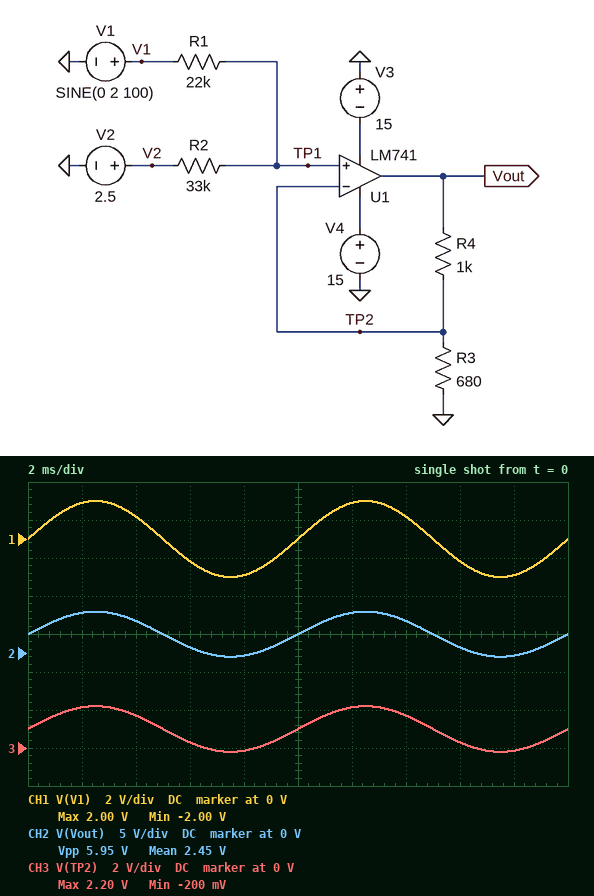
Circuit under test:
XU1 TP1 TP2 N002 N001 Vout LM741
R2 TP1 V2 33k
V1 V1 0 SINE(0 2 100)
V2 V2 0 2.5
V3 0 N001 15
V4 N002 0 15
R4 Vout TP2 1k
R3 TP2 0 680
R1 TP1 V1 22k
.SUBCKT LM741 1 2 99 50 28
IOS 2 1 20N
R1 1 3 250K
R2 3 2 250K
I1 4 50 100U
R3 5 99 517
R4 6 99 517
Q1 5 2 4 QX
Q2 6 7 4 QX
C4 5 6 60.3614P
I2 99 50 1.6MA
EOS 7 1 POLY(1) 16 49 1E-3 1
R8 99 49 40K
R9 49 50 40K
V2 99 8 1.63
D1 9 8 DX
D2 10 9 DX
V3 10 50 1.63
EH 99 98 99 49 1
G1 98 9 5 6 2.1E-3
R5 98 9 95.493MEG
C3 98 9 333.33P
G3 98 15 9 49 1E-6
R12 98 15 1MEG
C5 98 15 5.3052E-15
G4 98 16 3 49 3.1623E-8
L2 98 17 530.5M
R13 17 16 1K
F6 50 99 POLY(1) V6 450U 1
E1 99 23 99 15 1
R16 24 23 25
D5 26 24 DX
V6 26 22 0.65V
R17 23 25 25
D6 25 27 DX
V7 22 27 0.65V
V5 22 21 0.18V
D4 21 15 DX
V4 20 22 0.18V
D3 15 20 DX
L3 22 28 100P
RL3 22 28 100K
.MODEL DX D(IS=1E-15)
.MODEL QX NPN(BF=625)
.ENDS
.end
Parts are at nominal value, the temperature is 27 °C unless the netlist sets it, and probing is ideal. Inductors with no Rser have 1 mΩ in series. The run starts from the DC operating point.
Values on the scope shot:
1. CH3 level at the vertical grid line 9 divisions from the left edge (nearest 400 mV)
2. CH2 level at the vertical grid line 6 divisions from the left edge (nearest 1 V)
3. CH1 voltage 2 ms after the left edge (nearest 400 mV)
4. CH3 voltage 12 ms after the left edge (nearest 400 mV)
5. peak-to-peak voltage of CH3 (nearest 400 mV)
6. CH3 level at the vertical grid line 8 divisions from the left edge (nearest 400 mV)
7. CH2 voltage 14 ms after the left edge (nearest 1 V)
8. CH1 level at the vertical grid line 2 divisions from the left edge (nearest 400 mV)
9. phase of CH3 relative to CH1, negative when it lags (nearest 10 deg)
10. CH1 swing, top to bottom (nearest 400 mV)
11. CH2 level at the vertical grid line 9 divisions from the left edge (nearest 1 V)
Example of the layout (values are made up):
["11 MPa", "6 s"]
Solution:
["0 V", "5 V", "2.0 V", "2.0 V", "2.4 V", "400 mV", "4 V", "1.2 V", "0 deg", "4.0 V", "0 V"]
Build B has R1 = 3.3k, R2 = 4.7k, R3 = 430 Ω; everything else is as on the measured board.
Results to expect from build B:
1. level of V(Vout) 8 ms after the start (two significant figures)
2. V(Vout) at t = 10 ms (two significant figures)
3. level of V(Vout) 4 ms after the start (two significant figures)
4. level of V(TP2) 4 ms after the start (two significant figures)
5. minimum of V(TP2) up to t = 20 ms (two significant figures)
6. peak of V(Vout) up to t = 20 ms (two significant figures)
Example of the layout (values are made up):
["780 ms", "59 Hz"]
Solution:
["-280 mV", "3.4 V", "5.7 V", "1.7 V", "-140 mV", "7.3 V"]
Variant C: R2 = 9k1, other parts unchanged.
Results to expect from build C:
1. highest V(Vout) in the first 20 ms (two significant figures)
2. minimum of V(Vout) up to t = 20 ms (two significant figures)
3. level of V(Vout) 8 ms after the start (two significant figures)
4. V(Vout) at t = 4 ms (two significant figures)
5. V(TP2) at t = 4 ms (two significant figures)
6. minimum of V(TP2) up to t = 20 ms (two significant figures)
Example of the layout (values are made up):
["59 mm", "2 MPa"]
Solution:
["5.8 V", "2.9 V", "3.0 V", "5.2 V", "2.1 V", "1.2 V"]
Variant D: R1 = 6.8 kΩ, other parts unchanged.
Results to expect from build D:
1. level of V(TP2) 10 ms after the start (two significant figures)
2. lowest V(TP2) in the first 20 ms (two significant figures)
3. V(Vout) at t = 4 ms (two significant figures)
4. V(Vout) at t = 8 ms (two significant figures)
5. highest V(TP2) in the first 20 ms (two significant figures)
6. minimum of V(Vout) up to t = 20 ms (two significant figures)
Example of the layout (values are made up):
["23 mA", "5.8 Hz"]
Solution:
["430 mV", "-1.2 V", "3.5 V", "-2.8 V", "2.1 V", "-3.0 V"]
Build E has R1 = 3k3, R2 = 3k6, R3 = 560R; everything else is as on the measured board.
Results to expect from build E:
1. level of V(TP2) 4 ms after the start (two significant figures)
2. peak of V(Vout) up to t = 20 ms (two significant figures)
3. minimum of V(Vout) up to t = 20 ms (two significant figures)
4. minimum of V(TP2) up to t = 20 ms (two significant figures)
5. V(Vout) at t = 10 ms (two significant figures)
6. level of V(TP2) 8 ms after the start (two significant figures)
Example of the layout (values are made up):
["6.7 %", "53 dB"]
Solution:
["1.8 V", "6.2 V", "430 mV", "150 mV", "3.3 V", "200 mV"]
